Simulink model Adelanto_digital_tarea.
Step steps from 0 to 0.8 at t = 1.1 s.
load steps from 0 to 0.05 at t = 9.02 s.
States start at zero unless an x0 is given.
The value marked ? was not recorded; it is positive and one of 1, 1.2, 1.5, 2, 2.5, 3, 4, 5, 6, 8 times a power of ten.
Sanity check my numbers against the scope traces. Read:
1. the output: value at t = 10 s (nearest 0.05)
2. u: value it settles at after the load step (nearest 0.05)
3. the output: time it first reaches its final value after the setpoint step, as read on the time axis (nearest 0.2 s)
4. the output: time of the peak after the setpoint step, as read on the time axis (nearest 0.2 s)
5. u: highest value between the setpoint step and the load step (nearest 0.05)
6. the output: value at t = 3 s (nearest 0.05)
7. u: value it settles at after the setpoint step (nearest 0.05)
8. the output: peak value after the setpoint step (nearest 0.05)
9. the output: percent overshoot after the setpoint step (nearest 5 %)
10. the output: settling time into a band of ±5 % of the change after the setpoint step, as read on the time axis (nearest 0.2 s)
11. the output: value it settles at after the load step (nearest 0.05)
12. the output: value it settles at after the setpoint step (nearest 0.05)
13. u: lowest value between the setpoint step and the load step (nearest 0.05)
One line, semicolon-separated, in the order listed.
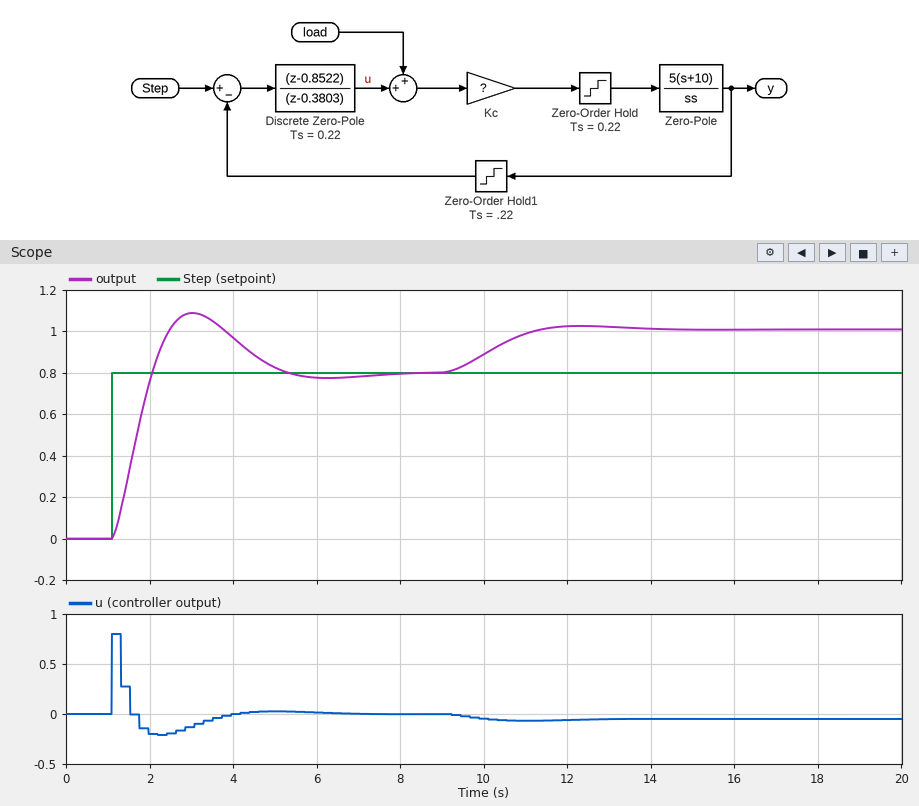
0.90; -0.05; 2.0 s; 3.0 s; 0.80; 1.10; 0.00; 1.10; 35 %; 4.8 s; 1.00; 0.80; -0.20
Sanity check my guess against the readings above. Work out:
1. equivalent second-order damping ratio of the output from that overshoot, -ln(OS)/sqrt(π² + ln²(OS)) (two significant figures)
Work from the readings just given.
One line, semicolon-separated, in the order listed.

0.32
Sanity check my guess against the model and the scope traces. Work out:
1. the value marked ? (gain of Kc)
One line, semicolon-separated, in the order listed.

0.08
